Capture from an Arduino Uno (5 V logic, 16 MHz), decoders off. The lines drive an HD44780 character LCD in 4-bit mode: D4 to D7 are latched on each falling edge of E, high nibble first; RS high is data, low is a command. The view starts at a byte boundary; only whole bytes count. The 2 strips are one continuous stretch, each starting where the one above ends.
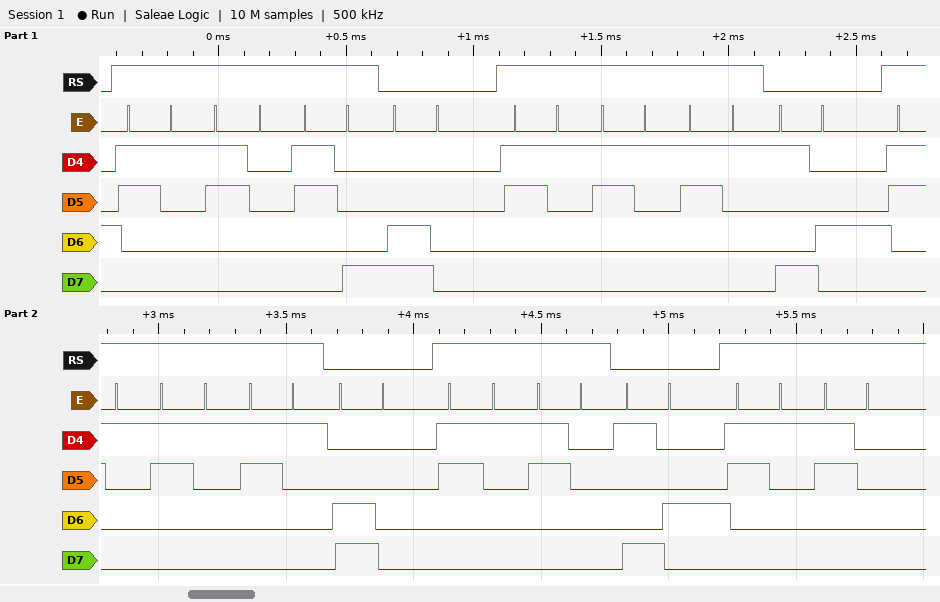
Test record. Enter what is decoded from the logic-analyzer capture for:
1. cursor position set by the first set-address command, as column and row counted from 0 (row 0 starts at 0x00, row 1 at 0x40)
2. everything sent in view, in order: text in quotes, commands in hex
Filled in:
column 0, row 1
"108" 0xC0 "111" 0x94 "111" 0xC0 "10" 0x94 "10"
